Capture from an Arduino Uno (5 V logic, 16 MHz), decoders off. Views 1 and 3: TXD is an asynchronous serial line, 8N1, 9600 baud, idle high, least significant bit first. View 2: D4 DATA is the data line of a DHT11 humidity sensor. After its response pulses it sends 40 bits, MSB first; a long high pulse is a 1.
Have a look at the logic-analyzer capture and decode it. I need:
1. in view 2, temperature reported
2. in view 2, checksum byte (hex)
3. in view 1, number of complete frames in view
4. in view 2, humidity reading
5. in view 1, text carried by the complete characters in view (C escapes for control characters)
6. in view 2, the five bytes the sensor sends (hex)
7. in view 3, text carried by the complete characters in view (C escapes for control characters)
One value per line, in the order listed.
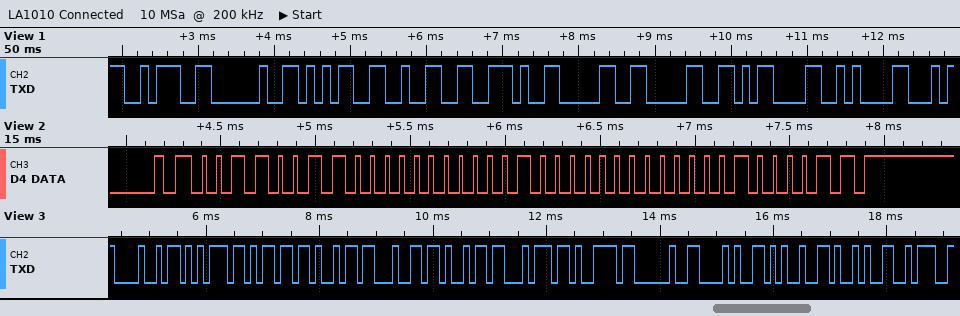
16.0 °C
0x43
9
51 %
": 52.00\r\n"
33 00 10 00 43
"Humidity (%):"
